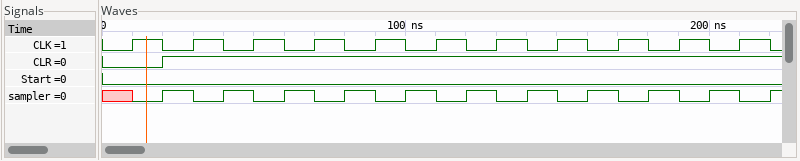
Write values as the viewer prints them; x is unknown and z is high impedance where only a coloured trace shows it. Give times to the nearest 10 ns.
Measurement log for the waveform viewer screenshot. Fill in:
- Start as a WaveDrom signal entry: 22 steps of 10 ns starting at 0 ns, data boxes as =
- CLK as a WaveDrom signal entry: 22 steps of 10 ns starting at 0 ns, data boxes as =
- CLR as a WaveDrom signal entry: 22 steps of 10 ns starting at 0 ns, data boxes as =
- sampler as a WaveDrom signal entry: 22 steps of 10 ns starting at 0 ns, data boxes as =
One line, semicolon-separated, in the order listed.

{name: 'Start', wave: '0.....................'}; {name: 'CLK', wave: '0101010101010101010101'}; {name: 'CLR', wave: '0.1...................'}; {name: 'sampler', wave: 'x010101010101010101010'}
